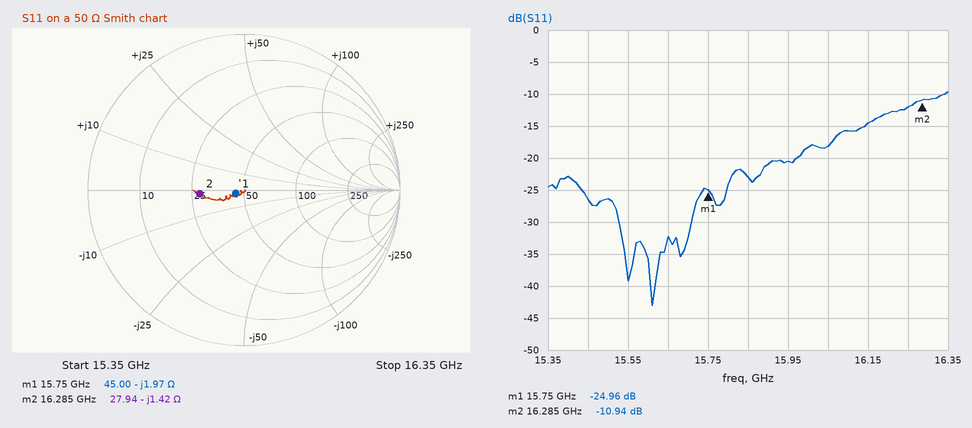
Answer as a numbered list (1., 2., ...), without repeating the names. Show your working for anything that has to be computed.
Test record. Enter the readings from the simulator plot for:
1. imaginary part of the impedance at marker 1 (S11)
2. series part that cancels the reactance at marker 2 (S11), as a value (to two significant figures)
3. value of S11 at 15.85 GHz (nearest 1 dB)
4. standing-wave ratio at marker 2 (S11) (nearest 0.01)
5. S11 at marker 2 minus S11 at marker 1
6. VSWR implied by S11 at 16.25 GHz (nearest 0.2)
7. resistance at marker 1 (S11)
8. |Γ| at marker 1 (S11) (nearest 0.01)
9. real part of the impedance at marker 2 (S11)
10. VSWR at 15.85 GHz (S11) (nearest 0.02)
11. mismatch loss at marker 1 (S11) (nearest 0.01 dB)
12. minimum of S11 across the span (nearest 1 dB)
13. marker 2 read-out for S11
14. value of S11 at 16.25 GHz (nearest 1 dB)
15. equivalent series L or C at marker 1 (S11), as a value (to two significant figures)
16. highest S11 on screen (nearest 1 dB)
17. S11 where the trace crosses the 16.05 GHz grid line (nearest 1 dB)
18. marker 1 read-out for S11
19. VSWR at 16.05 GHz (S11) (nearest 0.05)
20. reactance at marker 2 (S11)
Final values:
1. -1.97 Ω
2. L = 1.42 Ω/(2π × 16.285 GHz) ≈ 14 pH
3. -23 dB
4. 1.79
5. -10.94 − (-24.96) = 14.02 dB
6. |Γ| = 10^(-12/20) = 0.2512; VSWR = (1 + 0.2512)/(1 − 0.2512) ≈ 1.67, so 1.6 to the nearest 0.2
7. 45.00 Ω
8. 0.06
9. 27.94 Ω
10. |Γ| = 10^(-23/20) = 0.0708; VSWR = (1 + 0.0708)/(1 − 0.0708) ≈ 1.15, so 1.16 to the nearest 0.02
11. −10 log10(1 − 10^(-24.96/10)) ≈ 0.01 dB
12. -43 dB
13. -10.94 dB
14. -12 dB
15. C = 1/(2π × 15.75 GHz × 1.97 Ω) ≈ 5.1 pF
16. -10 dB
17. -18 dB
18. -24.96 dB
19. |Γ| = 10^(-18/20) = 0.1259; VSWR = (1 + 0.1259)/(1 − 0.1259) ≈ 1.29, so 1.30 to the nearest 0.05
20. -1.42 Ω
